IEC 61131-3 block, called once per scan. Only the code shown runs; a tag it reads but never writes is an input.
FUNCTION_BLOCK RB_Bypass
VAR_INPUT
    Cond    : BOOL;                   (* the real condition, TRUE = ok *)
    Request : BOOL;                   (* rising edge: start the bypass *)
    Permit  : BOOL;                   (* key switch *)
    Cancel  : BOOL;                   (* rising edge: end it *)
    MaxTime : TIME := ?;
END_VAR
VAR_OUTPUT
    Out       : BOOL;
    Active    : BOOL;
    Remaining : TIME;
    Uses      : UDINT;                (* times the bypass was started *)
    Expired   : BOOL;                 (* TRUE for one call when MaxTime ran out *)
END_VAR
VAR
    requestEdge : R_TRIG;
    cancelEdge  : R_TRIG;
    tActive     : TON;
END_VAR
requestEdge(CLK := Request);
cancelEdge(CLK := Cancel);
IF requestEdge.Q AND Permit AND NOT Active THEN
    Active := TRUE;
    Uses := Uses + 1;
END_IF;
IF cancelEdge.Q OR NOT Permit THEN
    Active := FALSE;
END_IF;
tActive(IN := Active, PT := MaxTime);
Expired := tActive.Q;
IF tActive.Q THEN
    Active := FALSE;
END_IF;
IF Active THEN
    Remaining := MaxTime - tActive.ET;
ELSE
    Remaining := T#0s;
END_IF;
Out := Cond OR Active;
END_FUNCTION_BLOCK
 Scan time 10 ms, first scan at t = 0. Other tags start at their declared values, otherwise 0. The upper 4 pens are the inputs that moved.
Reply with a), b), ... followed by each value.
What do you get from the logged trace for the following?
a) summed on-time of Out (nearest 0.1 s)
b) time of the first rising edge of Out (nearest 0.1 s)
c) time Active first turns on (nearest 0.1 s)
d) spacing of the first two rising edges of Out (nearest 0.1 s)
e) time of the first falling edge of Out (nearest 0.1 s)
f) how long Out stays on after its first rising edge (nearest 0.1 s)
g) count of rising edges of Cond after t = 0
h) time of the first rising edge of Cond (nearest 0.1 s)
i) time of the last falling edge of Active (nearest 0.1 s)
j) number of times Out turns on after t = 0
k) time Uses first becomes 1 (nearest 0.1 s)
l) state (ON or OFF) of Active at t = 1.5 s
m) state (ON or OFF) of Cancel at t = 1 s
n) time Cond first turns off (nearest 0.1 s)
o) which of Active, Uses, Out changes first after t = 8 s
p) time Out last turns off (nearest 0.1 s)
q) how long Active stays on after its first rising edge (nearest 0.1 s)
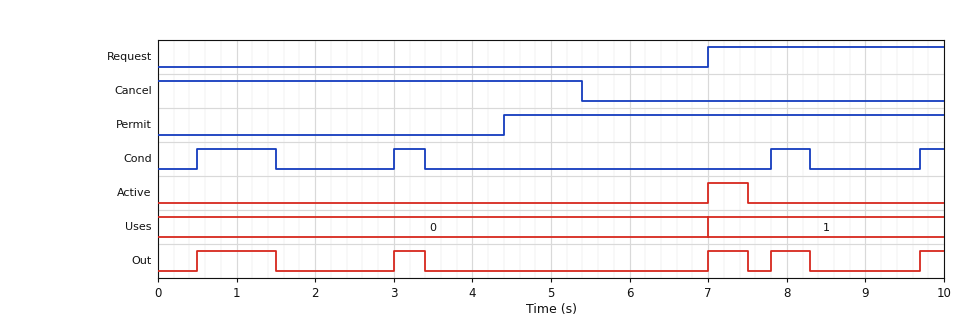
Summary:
a) 2.7 s
b) 0.5 s
c) 7.0 s
d) 2.5 s
e) 1.5 s
f) 1.0 s
g) 4
h) 0.5 s
i) 7.5 s
j) 5
k) 7.0 s
l) OFF
m) ON
n) 1.5 s
o) Out
p) 8.3 s
q) 0.5 s
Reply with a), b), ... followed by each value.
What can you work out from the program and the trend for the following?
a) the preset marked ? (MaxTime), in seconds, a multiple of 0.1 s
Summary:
a) 0.5 s
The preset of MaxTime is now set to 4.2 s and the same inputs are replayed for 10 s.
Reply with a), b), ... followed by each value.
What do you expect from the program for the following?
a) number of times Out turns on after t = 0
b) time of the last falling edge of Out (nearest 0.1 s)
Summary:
a) 3
b) 3.4 s
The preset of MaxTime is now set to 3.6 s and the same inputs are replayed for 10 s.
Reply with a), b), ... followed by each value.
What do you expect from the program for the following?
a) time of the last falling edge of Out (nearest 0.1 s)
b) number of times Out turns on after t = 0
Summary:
a) 3.4 s
b) 3
